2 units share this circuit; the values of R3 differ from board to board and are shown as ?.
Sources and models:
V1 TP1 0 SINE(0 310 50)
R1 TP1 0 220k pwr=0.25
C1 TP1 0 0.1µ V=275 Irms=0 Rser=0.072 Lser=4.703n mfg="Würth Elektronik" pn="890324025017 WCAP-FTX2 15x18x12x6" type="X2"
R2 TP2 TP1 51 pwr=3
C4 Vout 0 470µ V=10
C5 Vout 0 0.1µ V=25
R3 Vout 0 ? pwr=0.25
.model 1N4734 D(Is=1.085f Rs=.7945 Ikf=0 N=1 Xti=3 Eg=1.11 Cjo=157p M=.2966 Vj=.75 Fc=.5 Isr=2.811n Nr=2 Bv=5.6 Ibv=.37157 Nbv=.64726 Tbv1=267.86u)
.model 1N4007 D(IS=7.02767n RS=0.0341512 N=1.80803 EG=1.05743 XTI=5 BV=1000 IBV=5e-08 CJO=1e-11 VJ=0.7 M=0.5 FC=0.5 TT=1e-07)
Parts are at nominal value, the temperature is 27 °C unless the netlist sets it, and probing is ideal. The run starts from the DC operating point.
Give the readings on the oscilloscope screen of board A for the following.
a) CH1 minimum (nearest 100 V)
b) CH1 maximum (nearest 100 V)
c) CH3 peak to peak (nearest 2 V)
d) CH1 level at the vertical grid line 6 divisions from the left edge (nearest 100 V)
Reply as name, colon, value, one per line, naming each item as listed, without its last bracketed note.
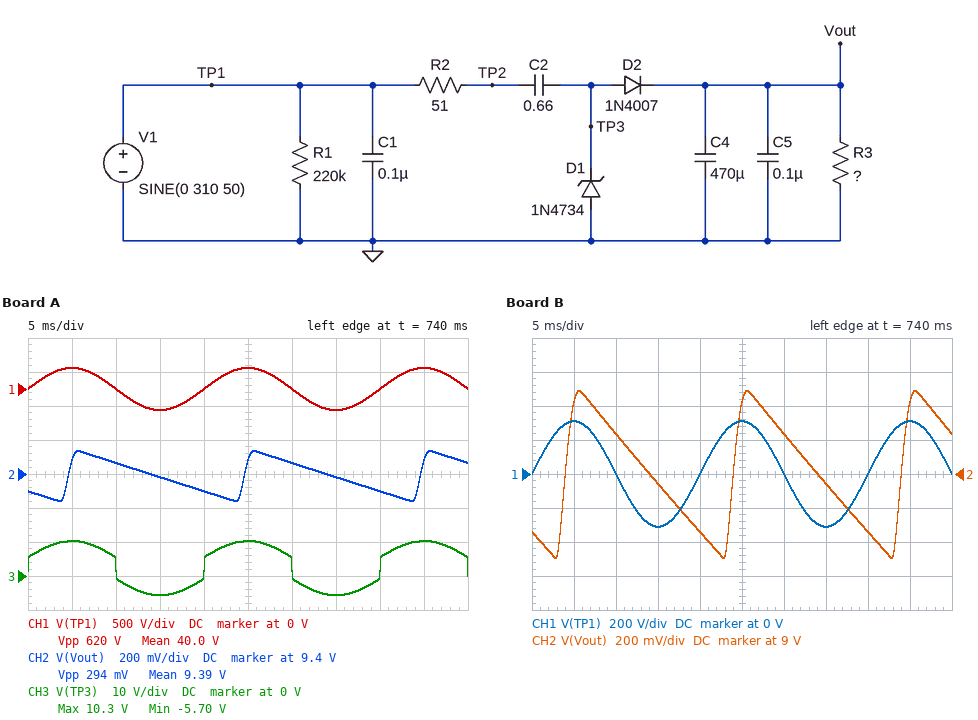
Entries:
CH1 minimum: -300 V
CH1 maximum: 300 V
CH3 peak to peak: 16 V
CH1 level at the vertical grid line 6 divisions from the left edge: 0 V
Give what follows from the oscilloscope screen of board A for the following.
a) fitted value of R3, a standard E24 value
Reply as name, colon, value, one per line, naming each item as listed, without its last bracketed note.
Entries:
fitted value of R3, a standard E24 value: 1.2 kΩ
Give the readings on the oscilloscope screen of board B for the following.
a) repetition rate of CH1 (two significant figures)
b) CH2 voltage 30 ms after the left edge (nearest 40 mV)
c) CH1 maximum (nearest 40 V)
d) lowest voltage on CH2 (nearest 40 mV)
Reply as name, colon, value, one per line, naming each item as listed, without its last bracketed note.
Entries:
repetition rate of CH1: 50 Hz
CH2 voltage 30 ms after the left edge: 9.24 V
CH1 maximum: 320 V
lowest voltage on CH2: 8.52 V
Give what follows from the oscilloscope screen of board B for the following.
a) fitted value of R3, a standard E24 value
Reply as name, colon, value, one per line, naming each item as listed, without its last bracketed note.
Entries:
fitted value of R3, a standard E24 value: 330 Ω
